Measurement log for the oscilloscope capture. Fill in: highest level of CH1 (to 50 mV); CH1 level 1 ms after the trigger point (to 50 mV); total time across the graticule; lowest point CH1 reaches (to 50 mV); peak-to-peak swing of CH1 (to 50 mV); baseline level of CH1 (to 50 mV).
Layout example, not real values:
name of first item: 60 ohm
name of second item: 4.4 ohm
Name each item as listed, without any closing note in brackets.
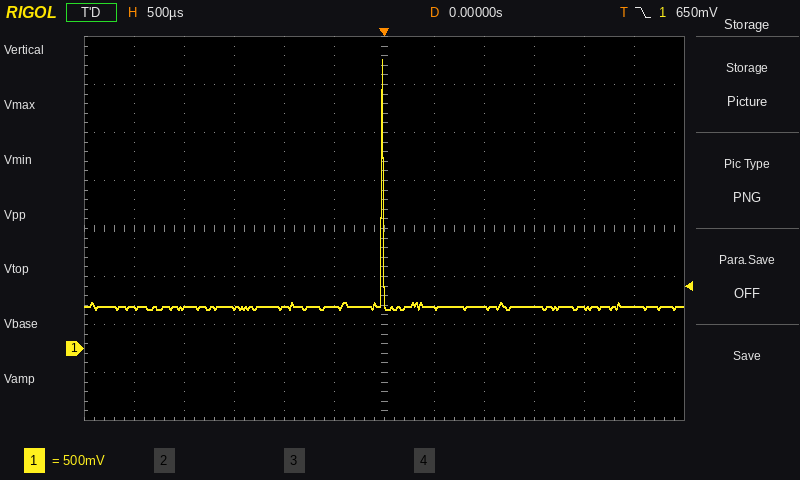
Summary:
highest level of CH1: 3.00 V
CH1 level 1 ms after the trigger point: 450 mV
total time across the graticule: 6 ms
lowest point CH1 reaches: 400 mV
peak-to-peak swing of CH1: 2.60 V
baseline level of CH1: 450 mV
